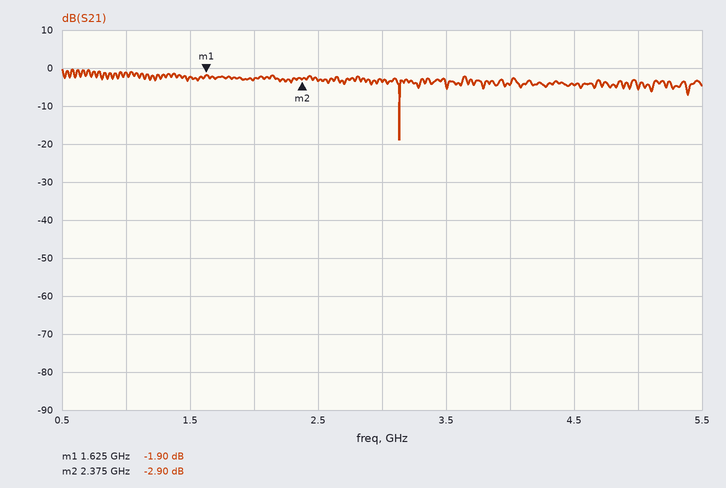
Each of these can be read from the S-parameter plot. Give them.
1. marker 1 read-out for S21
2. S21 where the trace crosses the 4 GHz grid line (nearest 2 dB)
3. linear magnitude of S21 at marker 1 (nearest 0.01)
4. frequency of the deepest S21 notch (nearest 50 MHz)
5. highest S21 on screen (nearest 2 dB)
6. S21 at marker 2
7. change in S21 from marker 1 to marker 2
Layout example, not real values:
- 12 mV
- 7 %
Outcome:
- -1.90 dB
- -4 dB
- 0.80
- 3.15 GHz
- 0 dB
- -2.90 dB
- -1.00 dB
